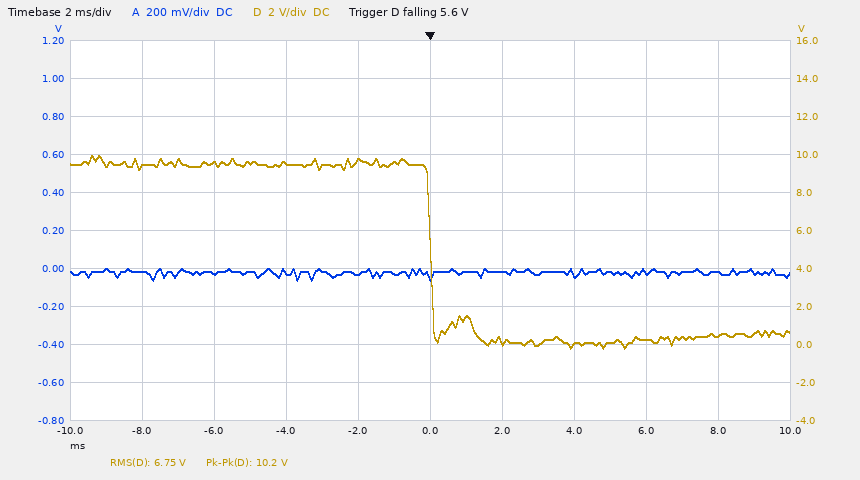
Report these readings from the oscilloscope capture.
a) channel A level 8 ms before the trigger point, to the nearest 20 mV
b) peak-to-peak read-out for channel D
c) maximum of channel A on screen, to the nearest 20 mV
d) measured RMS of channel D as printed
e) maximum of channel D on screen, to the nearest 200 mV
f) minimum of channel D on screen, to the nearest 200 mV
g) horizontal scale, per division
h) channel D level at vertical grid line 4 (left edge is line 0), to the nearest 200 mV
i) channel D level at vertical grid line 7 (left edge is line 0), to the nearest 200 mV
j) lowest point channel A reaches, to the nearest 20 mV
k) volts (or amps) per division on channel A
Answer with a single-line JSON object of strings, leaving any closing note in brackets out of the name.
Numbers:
{"channel A level 8 ms before the trigger point, to the nearest 20 mV": "-20 mV", "peak-to-peak read-out for channel D": "10.2 V", "maximum of channel A on screen, to the nearest 20 mV": "0 mV", "measured RMS of channel D as printed": "6.75 V", "maximum of channel D on screen, to the nearest 200 mV": "10.0 V", "minimum of channel D on screen, to the nearest 200 mV": "-200 mV", "horizontal scale, per division": "2 ms", "channel D level at vertical grid line 4 (left edge is line 0), to the nearest 200 mV": "9.6 V", "channel D level at vertical grid line 7 (left edge is line 0), to the nearest 200 mV": "0.0 V", "lowest point channel A reaches, to the nearest 20 mV": "-60 mV", "volts (or amps) per division on channel A": "200 mV"}
